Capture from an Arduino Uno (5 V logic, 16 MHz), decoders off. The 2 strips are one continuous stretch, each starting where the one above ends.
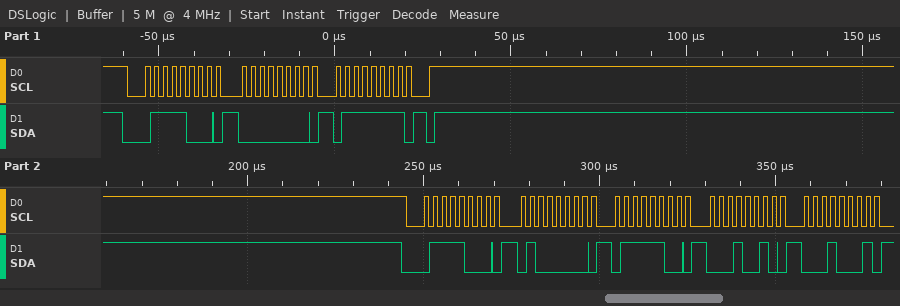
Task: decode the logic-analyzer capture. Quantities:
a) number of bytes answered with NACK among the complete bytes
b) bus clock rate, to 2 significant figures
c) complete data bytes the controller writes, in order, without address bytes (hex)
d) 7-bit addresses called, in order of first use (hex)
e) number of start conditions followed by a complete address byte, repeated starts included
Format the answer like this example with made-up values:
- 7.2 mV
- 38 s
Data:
- 0
- 400 kHz
- 00 7F 40 7C 12 11
- 0x3C
- 2
